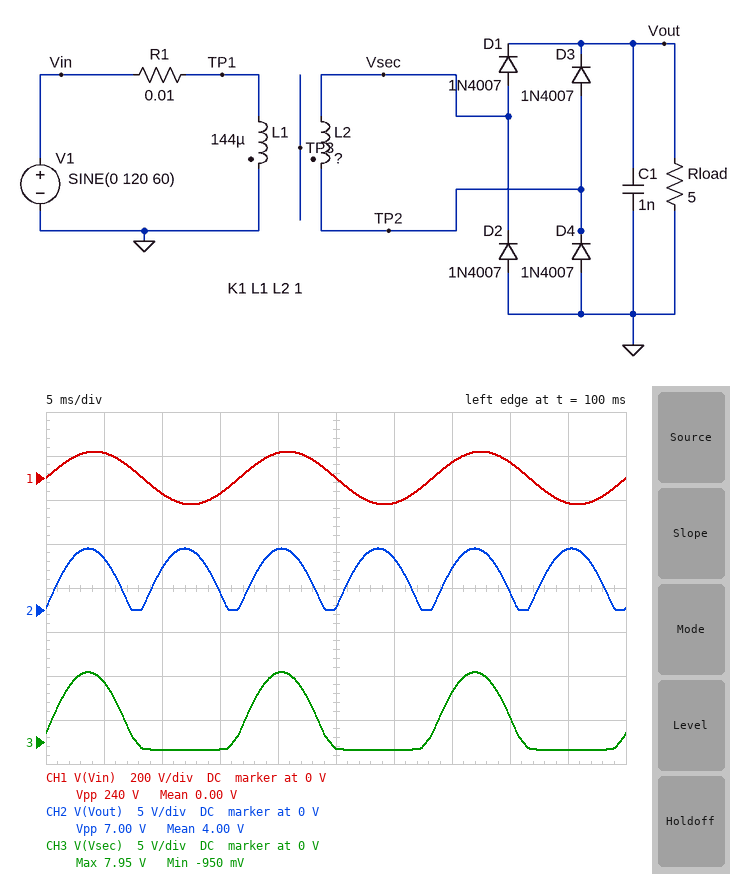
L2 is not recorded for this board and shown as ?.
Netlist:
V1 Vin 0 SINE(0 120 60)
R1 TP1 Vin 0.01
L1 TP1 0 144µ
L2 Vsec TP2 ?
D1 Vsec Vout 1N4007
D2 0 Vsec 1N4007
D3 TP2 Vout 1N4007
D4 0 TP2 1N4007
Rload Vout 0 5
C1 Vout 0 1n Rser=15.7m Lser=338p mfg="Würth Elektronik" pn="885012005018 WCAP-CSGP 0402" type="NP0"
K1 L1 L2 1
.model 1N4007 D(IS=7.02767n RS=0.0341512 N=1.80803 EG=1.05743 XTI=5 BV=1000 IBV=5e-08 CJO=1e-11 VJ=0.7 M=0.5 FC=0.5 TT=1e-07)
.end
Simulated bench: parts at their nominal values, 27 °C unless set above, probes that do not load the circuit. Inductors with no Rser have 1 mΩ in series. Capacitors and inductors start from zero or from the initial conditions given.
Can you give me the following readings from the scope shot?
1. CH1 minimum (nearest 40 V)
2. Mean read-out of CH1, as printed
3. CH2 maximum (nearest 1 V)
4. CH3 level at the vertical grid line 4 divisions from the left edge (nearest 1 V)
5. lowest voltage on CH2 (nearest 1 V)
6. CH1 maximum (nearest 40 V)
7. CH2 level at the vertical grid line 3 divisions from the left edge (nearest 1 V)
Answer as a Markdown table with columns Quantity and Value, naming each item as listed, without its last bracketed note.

| Quantity | Value |
|---|---|
| CH1 minimum | -120 V |
| Mean read-out of CH1, as printed | 0.00 V |
| CH2 maximum | 7 V |
| CH3 level at the vertical grid line 4 divisions from the left edge | 8 V |
| lowest voltage on CH2 | 0 V |
| CH1 maximum | 120 V |
| CH2 level at the vertical grid line 3 divisions from the left edge | 2 V |
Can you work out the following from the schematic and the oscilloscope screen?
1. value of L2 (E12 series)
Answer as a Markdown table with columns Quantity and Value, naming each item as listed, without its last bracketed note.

| Quantity | Value |
|---|---|
| value of L2 | 820 nH |
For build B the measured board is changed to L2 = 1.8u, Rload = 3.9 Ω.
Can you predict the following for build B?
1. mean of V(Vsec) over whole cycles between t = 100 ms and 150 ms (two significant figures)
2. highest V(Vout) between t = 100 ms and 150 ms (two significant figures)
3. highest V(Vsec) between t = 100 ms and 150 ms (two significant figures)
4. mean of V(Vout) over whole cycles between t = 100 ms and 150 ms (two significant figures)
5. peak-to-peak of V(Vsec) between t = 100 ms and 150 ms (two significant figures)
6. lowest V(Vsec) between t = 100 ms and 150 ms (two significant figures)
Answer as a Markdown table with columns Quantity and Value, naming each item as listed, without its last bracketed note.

| Quantity | Value |
|---|---|
| mean of V(Vsec) over whole cycles between t = 100 ms and 150 ms | 3.3 V |
| highest V(Vout) between t = 100 ms and 150 ms | 11 V |
| highest V(Vsec) between t = 100 ms and 150 ms | 12 V |
| mean of V(Vout) over whole cycles between t = 100 ms and 150 ms | 6.5 V |
| peak-to-peak of V(Vsec) between t = 100 ms and 150 ms | 13 V |
| lowest V(Vsec) between t = 100 ms and 150 ms | -1.0 V |
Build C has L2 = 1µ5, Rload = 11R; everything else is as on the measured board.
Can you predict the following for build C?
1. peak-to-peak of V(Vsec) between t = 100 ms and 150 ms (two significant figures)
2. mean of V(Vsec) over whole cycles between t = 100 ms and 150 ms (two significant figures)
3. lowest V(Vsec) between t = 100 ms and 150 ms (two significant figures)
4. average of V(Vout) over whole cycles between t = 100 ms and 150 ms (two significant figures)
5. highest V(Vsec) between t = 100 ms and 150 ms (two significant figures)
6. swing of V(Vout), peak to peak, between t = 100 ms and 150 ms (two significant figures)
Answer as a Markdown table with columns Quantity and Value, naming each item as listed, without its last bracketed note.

| Quantity | Value |
|---|---|
| peak-to-peak of V(Vsec) between t = 100 ms and 150 ms | 12 V |
| mean of V(Vsec) over whole cycles between t = 100 ms and 150 ms | 3.0 V |
| lowest V(Vsec) between t = 100 ms and 150 ms | -910 mV |
| average of V(Vout) over whole cycles between t = 100 ms and 150 ms | 6.0 V |
| highest V(Vsec) between t = 100 ms and 150 ms | 11 V |
| swing of V(Vout), peak to peak, between t = 100 ms and 150 ms | 10 V |
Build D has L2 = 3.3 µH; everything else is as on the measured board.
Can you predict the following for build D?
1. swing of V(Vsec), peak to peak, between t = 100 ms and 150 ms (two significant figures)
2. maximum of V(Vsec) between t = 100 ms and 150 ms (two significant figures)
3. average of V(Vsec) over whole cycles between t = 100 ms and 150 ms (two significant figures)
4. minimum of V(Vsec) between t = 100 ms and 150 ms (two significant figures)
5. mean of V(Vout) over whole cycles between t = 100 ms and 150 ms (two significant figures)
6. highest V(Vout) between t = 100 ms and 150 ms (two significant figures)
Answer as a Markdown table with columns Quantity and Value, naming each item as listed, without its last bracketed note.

| Quantity | Value |
|---|---|
| swing of V(Vsec), peak to peak, between t = 100 ms and 150 ms | 18 V |
| maximum of V(Vsec) between t = 100 ms and 150 ms | 17 V |
| average of V(Vsec) over whole cycles between t = 100 ms and 150 ms | 4.7 V |
| minimum of V(Vsec) between t = 100 ms and 150 ms | -1.0 V |
| mean of V(Vout) over whole cycles between t = 100 ms and 150 ms | 9.5 V |
| highest V(Vout) between t = 100 ms and 150 ms | 16 V |
